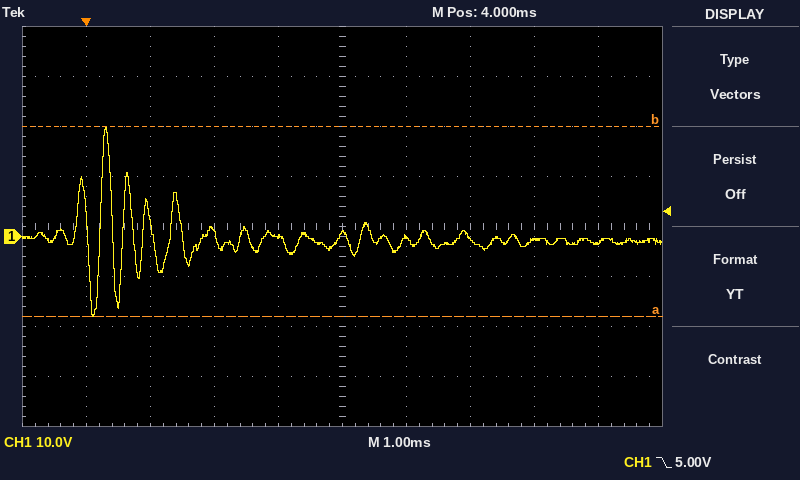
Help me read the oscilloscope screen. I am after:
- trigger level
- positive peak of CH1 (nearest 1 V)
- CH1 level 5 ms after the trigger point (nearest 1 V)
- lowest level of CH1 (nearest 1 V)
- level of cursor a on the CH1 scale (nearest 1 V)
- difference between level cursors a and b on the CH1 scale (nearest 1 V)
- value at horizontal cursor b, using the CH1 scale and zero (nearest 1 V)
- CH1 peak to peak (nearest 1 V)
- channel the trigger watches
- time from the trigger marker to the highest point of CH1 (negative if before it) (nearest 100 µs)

5.00 V
22 V
0 V
-16 V
-16 V
38 V
22 V
38 V
CH1
+300 µs
